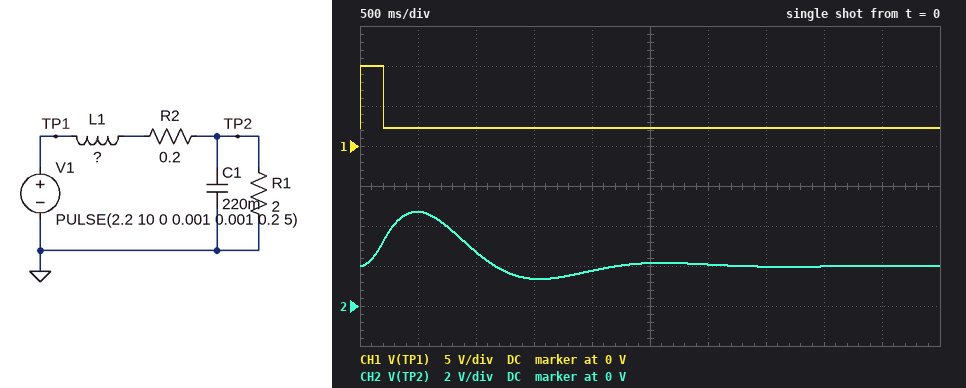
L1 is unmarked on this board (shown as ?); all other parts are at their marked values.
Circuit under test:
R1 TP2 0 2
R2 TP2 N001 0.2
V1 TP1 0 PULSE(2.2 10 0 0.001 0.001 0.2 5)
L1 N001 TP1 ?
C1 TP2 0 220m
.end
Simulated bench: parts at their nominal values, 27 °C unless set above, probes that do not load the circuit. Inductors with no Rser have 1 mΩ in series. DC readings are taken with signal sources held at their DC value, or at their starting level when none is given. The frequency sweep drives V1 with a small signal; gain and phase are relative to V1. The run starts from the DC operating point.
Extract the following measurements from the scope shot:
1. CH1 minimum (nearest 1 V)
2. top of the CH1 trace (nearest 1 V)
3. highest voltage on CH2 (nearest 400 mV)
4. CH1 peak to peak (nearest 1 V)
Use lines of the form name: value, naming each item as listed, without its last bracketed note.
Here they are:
CH1 minimum: 2 V
top of the CH1 trace: 10 V
highest voltage on CH2: 4.8 V
CH1 peak to peak: 8 V
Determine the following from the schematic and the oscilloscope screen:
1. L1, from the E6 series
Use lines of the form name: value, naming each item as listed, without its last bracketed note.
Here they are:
L1, from the E6 series: 470 mH
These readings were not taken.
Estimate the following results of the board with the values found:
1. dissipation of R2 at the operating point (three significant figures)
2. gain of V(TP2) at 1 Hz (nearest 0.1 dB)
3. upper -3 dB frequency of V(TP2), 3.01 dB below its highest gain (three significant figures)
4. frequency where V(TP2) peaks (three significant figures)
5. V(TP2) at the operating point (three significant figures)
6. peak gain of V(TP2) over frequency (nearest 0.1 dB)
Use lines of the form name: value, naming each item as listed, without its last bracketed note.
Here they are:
dissipation of R2 at the operating point: 200 mW
gain of V(TP2) at 1 Hz: -10.8 dB
upper -3 dB frequency of V(TP2), 3.01 dB below its highest gain: 617 mHz
frequency where V(TP2) peaks: 421 mHz
V(TP2) at the operating point: 2.00 V
peak gain of V(TP2) over frequency: 1.6 dB
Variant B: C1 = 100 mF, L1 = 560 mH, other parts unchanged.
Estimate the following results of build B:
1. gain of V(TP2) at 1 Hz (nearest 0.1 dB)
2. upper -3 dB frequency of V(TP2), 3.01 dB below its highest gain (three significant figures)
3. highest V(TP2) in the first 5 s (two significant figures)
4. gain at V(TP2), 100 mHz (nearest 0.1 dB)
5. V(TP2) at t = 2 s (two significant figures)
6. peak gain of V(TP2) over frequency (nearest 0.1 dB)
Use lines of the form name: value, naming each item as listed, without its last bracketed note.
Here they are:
gain of V(TP2) at 1 Hz: -6.8 dB
upper -3 dB frequency of V(TP2), 3.01 dB below its highest gain: 783 mHz
highest V(TP2) in the first 5 s: 5.0 V
gain at V(TP2), 100 mHz: -0.8 dB
V(TP2) at t = 2 s: 2.0 V
peak gain of V(TP2) over frequency: -0.5 dB
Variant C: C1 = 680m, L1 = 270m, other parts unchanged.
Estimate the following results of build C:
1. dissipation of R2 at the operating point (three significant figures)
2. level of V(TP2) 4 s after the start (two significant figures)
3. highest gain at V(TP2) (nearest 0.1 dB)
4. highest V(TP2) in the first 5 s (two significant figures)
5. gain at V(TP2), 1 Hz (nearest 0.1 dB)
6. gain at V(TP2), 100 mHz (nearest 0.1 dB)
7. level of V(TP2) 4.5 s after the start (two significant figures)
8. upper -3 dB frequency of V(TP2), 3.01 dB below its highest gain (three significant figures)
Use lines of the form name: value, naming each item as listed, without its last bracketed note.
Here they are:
dissipation of R2 at the operating point: 200 mW
level of V(TP2) 4 s after the start: 2.1 V
highest gain at V(TP2): 4.0 dB
highest V(TP2) in the first 5 s: 4.3 V
gain at V(TP2), 1 Hz: -16.1 dB
gain at V(TP2), 100 mHz: -0.4 dB
level of V(TP2) 4.5 s after the start: 1.9 V
upper -3 dB frequency of V(TP2), 3.01 dB below its highest gain: 460 mHz
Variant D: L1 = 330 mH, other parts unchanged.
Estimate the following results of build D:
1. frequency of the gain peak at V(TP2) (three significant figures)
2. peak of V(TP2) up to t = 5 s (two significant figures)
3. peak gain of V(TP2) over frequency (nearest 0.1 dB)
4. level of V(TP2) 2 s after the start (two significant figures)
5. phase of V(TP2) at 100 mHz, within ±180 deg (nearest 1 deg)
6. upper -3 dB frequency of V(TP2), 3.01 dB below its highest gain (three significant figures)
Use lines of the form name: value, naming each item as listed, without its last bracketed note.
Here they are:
frequency of the gain peak at V(TP2): 528 mHz
peak of V(TP2) up to t = 5 s: 5.4 V
peak gain of V(TP2) over frequency: 2.4 dB
level of V(TP2) 2 s after the start: 2.2 V
phase of V(TP2) at 100 mHz, within ±180 deg: -7 deg
upper -3 dB frequency of V(TP2), 3.01 dB below its highest gain: 737 mHz
